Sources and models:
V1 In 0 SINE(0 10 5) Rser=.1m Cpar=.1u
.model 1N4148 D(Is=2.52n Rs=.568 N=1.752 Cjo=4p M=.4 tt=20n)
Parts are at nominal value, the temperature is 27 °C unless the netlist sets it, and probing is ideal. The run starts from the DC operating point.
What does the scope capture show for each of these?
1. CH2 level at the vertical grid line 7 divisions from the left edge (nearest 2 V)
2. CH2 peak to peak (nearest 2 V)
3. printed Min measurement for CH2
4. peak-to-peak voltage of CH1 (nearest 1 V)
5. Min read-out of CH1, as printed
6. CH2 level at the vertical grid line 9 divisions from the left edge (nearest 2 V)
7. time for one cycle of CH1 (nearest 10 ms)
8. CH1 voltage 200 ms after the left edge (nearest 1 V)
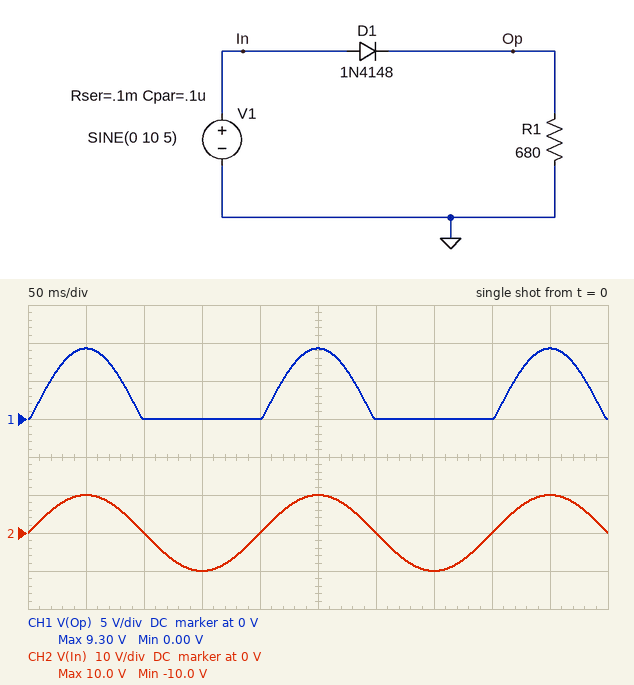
-10 V
20 V
-10.0 V
9 V
0.00 V
10 V
200 ms
0 V
